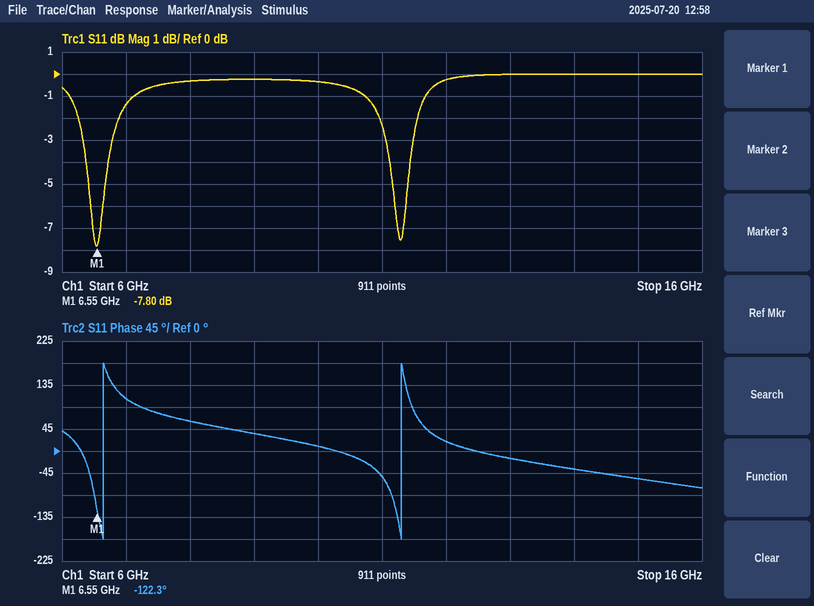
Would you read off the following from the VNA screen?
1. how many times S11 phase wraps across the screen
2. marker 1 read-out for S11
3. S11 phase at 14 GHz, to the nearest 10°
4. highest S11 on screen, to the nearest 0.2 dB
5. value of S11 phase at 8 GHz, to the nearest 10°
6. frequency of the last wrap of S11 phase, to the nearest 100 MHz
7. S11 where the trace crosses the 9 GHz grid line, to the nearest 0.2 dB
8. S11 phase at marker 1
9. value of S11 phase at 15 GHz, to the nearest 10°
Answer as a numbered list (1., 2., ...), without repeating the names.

1. 2
2. -7.80 dB
3. -40°
4. 0.0 dB
5. 60°
6. 11.3 GHz
7. -0.2 dB
8. -122.3°
9. -60°
